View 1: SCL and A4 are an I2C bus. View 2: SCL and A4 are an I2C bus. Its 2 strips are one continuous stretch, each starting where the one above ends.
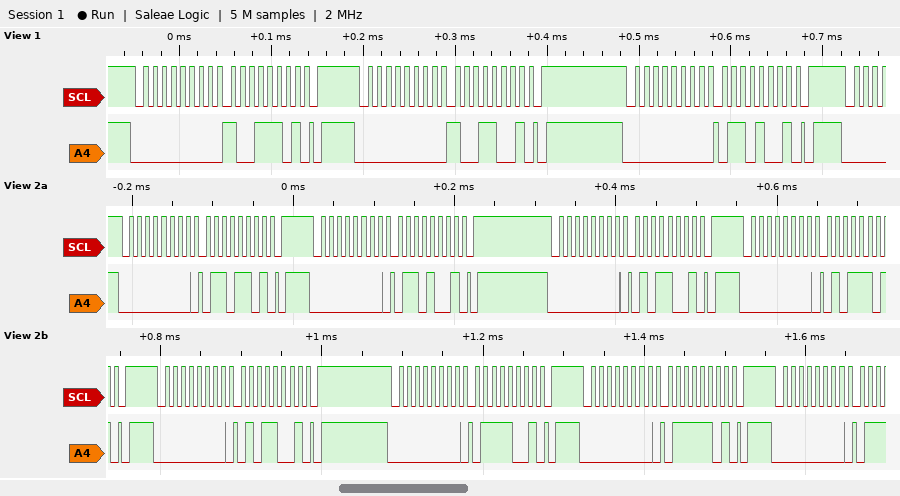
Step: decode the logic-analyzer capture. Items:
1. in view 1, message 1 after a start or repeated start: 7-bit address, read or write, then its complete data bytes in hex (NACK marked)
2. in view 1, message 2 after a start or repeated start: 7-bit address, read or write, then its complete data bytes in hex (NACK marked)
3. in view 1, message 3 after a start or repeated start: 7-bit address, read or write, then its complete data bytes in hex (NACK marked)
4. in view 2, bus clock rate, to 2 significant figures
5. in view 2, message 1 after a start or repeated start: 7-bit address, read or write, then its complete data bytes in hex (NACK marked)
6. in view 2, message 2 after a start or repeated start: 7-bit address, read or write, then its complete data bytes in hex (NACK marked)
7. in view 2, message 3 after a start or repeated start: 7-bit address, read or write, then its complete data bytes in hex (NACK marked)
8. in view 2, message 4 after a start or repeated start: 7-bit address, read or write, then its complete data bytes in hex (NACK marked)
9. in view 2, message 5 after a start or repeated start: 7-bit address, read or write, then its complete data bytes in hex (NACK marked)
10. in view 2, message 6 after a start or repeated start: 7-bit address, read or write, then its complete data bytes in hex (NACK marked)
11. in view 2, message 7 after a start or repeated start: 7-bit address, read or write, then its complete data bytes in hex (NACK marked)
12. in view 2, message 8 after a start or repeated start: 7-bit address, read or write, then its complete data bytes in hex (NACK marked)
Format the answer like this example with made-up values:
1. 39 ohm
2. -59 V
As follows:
1. 0x00 write: 9D
2. 0x00 write: 99
3. 0x00 write: 69
4. 100 kHz
5. 0x00 write: 6D
6. 0x00 write: 69
7. 0x00 write: 59
8. 0x00 write: 5D
9. 0x00 write: 59
10. 0x00 write: 79
11. 0x00 write: 7D
12. 0x00 write
